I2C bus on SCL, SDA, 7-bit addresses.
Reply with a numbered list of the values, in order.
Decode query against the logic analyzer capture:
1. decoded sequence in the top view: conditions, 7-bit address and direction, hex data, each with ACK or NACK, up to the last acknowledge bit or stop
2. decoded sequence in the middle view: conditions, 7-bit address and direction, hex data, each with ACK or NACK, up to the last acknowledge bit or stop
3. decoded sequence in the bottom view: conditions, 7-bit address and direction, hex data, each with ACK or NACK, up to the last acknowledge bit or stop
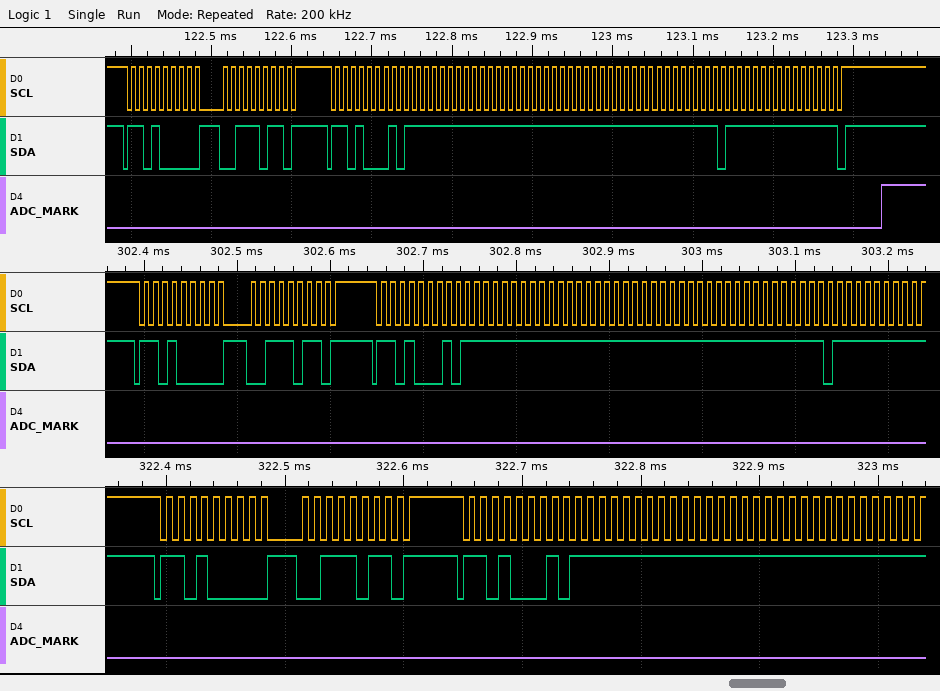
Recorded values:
1. start, address 68 write ACK, 3B ACK, repeated start, address 68 read ACK, FF NACK, FF NACK, FF NACK, FF NACK, EF NACK, FF NACK, stop
2. start, address 68 write ACK, 3B ACK, repeated start, address 68 read ACK, FF NACK, FF NACK, FF NACK, FF NACK, EF NACK
3. start, address 68 write ACK, 3B ACK, repeated start, address 68 read ACK, FF NACK, FF NACK, FF NACK
